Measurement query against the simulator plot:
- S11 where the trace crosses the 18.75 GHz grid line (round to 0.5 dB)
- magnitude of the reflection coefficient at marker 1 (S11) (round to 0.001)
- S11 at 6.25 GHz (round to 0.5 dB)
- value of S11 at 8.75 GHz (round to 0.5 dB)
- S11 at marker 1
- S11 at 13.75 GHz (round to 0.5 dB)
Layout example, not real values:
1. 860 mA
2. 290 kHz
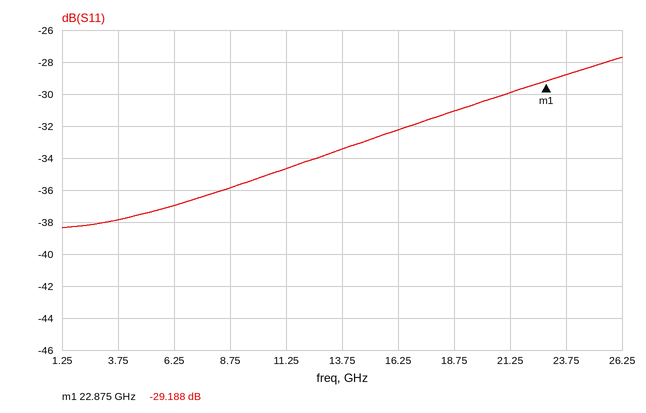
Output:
1. -31.0 dB
2. 0.035
3. -37.0 dB
4. -36.0 dB
5. -29.188 dB
6. -33.5 dB
